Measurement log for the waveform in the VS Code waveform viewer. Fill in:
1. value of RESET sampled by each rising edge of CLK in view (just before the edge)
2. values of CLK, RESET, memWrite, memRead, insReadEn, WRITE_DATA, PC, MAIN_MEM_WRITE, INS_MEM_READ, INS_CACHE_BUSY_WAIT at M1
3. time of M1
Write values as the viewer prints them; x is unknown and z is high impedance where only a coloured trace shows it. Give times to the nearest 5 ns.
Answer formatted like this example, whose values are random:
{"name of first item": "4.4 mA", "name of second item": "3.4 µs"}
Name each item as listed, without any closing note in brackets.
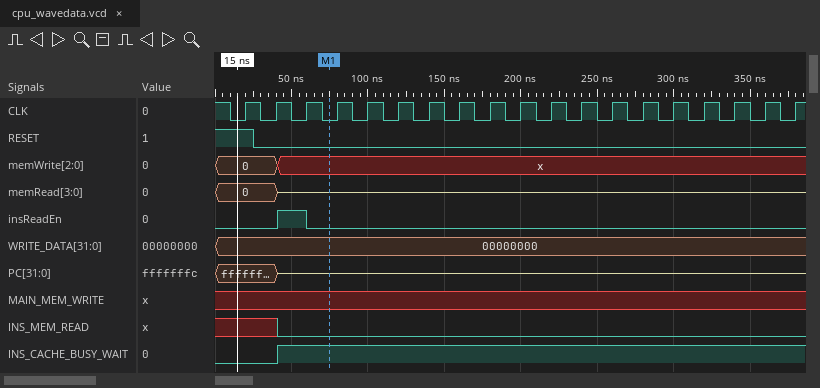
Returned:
{"value of RESET sampled by each rising edge of CLK in view": "1 0 0 0 0 0 0 0 0 0 0 0 0 0 0 0 0 0 0", "values of CLK, RESET, memWrite, memRead, insReadEn, WRITE_DATA, PC, MAIN_MEM_WRITE, INS_MEM_READ, INS_CACHE_BUSY_WAIT at M1": "CLK=0, RESET=0, memWrite=x, memRead=z, insReadEn=0, WRITE_DATA=00000000, PC=z, MAIN_MEM_WRITE=x, INS_MEM_READ=0, INS_CACHE_BUSY_WAIT=1", "time of M1": "75 ns"}
